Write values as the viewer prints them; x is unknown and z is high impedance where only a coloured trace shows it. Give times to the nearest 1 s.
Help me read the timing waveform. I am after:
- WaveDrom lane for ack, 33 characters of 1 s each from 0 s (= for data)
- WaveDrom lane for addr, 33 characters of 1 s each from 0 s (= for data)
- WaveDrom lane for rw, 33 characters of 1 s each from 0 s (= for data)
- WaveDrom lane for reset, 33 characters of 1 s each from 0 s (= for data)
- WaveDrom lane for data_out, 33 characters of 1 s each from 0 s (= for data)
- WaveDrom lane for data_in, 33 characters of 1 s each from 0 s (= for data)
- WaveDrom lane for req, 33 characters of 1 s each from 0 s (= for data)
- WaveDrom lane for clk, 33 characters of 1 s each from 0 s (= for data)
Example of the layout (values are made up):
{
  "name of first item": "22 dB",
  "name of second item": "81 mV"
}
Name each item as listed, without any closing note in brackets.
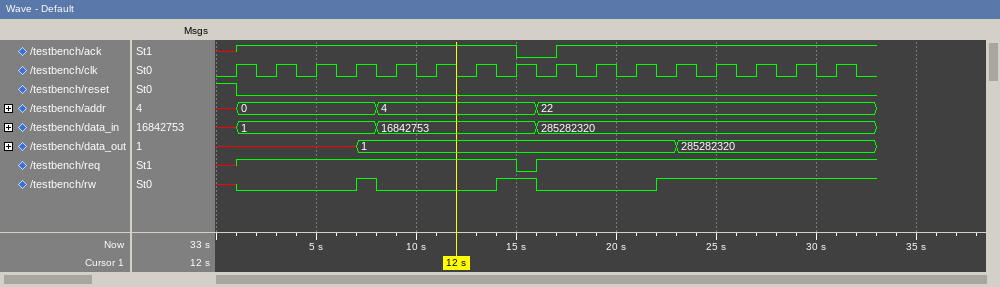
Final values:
{
  "WaveDrom lane for ack, 33 characters of 1 s each from 0 s": "{name: 'ack', wave: 'x1.............0.1...............'}",
  "WaveDrom lane for addr, 33 characters of 1 s each from 0 s": "{name: 'addr', wave: 'x=......=.......=................', data: '0 4 22'}",
  "WaveDrom lane for rw, 33 characters of 1 s each from 0 s": "{name: 'rw', wave: 'x0.....10.....1.0.....1..........'}",
  "WaveDrom lane for reset, 33 characters of 1 s each from 0 s": "{name: 'reset', wave: '10...............................'}",
  "WaveDrom lane for data_out, 33 characters of 1 s each from 0 s": "{name: 'data_out', wave: 'x......=...............=.........', data: '1 285282320'}",
  "WaveDrom lane for data_in, 33 characters of 1 s each from 0 s": "{name: 'data_in', wave: 'x=......=.......=................', data: '1 16842753 285282320'}",
  "WaveDrom lane for req, 33 characters of 1 s each from 0 s": "{name: 'req', wave: 'x1.............01................'}",
  "WaveDrom lane for clk, 33 characters of 1 s each from 0 s": "{name: 'clk', wave: '010101010101010101010101010101010'}"
}
